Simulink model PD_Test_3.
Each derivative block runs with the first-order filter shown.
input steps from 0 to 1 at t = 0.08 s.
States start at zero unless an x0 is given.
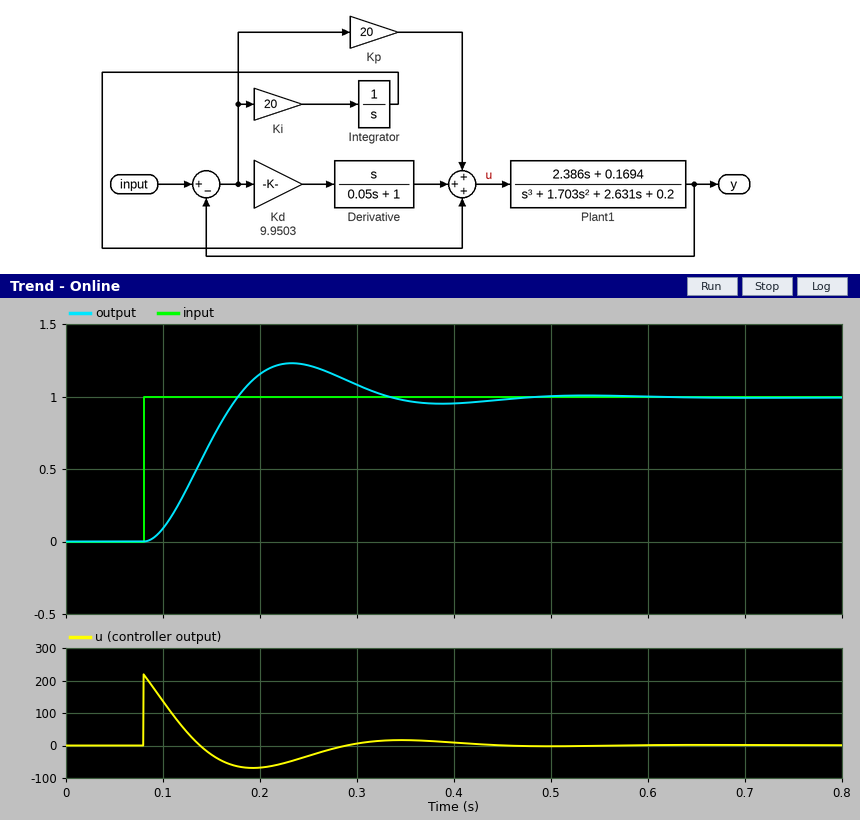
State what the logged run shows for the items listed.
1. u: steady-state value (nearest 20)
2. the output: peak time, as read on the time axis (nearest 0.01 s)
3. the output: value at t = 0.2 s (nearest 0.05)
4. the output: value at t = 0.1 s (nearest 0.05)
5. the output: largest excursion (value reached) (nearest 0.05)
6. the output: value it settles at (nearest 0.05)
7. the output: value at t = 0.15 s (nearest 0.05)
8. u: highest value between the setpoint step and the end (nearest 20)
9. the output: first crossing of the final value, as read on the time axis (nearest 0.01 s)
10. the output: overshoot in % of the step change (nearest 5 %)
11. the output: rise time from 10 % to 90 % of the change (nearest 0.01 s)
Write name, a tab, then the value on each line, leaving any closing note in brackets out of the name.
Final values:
u: steady-state value	0
the output: peak time, as read on the time axis	0.23 s
the output: value at t = 0.2 s	1.15
the output: value at t = 0.1 s	0.10
the output: largest excursion (value reached)	1.25
the output: value it settles at	1.00
the output: value at t = 0.15 s	0.70
u: highest value between the setpoint step and the end	220
the output: first crossing of the final value, as read on the time axis	0.18 s
the output: overshoot in % of the step change	25 %
the output: rise time from 10 % to 90 % of the change	0.07 s
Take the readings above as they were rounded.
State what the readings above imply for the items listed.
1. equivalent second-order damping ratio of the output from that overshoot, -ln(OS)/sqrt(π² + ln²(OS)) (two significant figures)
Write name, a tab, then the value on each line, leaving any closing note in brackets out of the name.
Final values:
equivalent second-order damping ratio of the output from that overshoot, -ln(OS)/sqrt(π² + ln²(OS))	0.40
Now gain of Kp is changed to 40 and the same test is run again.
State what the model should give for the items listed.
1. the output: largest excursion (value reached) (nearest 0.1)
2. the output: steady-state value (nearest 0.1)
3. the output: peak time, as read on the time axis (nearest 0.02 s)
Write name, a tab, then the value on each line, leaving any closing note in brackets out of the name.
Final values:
the output: largest excursion (value reached)	1.3
the output: steady-state value	1.0
the output: peak time, as read on the time axis	0.22 s
